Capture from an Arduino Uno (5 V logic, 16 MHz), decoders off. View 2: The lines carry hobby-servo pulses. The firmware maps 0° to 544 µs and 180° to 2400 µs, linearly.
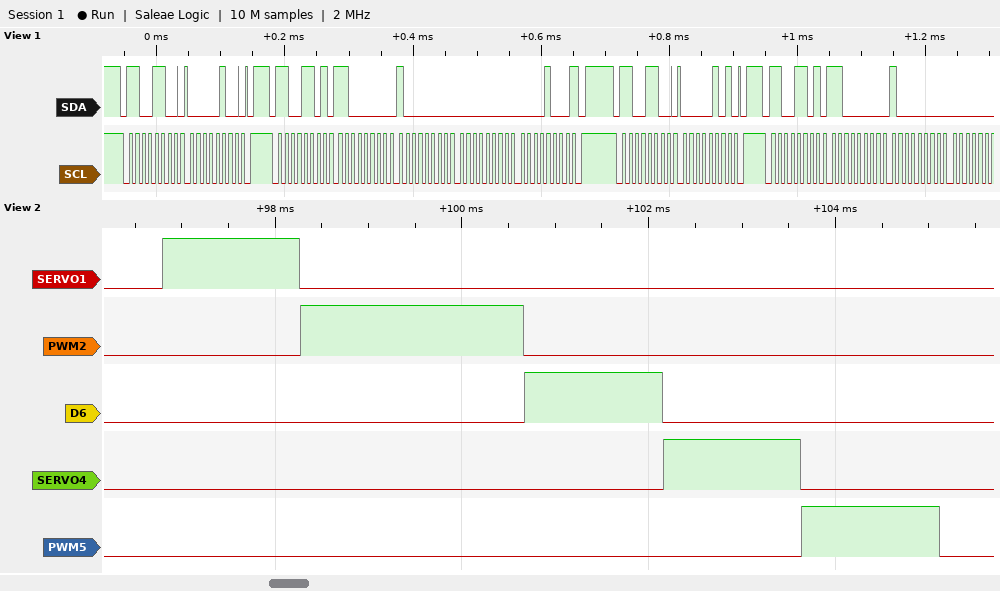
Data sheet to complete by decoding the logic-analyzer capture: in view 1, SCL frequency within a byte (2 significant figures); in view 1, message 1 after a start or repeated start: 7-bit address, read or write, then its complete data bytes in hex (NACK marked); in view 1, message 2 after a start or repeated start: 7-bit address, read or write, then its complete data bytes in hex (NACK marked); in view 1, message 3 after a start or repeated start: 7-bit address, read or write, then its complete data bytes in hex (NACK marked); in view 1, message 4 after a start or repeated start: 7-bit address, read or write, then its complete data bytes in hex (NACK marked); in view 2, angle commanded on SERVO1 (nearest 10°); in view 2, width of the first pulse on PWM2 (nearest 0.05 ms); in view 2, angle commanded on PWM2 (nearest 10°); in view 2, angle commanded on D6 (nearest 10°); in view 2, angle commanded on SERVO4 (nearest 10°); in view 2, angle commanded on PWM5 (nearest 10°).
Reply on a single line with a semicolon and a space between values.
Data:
100 kHz; 0x66 write: 04; 0x66 read: C0 80 00 08 NACK; 0x66 write: 05; 0x66 read: C0 80; 90°; 2.40 ms; 180°; 90°; 90°; 90°
